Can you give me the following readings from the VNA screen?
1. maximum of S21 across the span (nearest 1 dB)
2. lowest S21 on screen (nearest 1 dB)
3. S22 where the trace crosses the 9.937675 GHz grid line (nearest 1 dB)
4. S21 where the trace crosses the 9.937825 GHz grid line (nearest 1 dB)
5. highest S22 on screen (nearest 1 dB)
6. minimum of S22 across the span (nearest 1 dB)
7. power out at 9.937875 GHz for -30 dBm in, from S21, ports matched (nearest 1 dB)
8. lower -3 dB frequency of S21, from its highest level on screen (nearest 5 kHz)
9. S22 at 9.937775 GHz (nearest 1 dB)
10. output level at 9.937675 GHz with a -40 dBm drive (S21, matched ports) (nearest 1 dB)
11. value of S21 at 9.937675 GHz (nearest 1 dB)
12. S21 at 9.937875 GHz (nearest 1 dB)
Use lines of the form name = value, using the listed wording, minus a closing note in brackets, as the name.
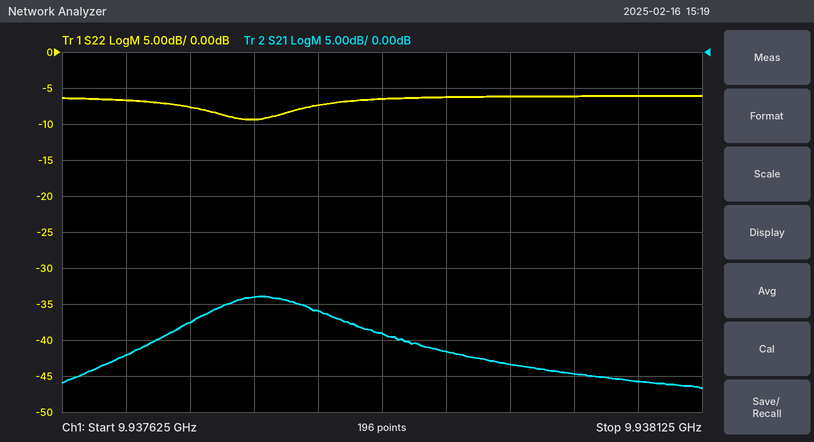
maximum of S21 across the span = -34 dB
lowest S21 on screen = -47 dB
S22 where the trace crosses the 9.937675 GHz grid line = -7 dB
S21 where the trace crosses the 9.937825 GHz grid line = -36 dB
highest S22 on screen = -6 dB
minimum of S22 across the span = -9 dB
power out at 9.937875 GHz for -30 dBm in, from S21, ports matched = -69 dBm
lower -3 dB frequency of S21, from its highest level on screen = 9.937730 GHz
S22 at 9.937775 GHz = -9 dB
output level at 9.937675 GHz with a -40 dBm drive (S21, matched ports) = -82 dBm
value of S21 at 9.937675 GHz = -42 dB
S21 at 9.937875 GHz = -39 dB
